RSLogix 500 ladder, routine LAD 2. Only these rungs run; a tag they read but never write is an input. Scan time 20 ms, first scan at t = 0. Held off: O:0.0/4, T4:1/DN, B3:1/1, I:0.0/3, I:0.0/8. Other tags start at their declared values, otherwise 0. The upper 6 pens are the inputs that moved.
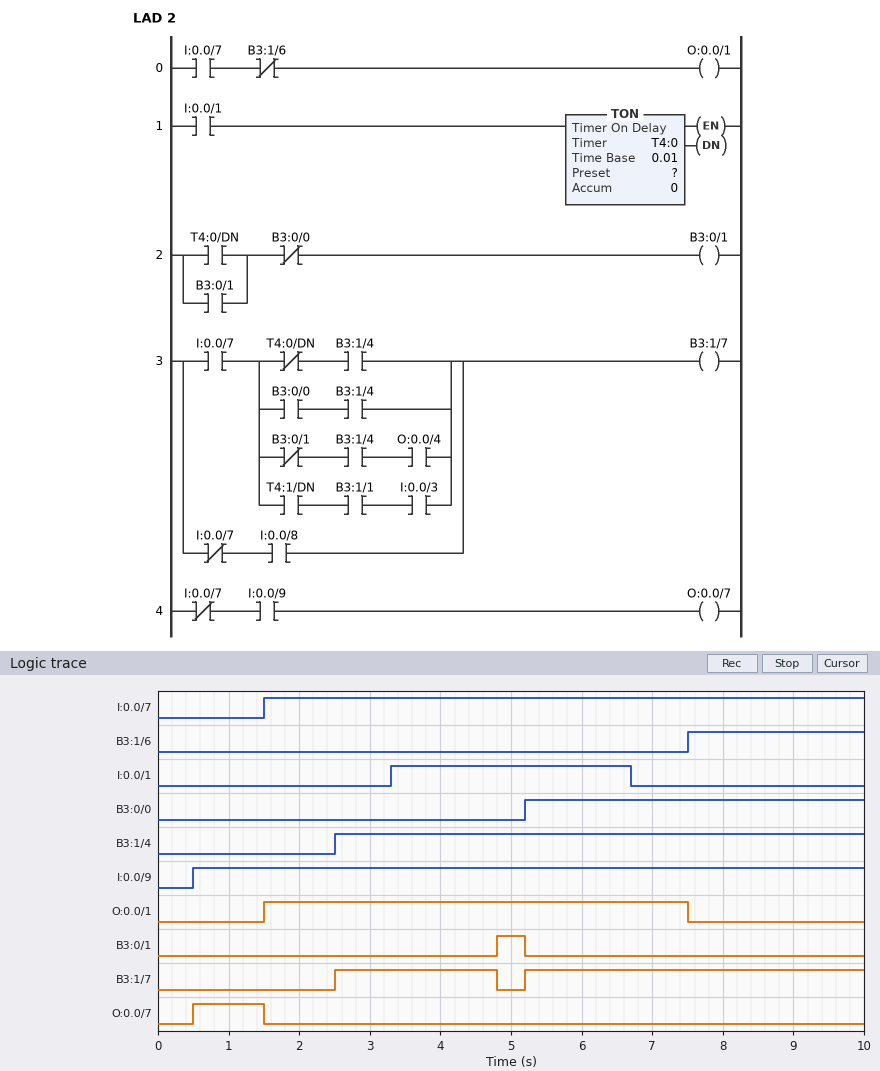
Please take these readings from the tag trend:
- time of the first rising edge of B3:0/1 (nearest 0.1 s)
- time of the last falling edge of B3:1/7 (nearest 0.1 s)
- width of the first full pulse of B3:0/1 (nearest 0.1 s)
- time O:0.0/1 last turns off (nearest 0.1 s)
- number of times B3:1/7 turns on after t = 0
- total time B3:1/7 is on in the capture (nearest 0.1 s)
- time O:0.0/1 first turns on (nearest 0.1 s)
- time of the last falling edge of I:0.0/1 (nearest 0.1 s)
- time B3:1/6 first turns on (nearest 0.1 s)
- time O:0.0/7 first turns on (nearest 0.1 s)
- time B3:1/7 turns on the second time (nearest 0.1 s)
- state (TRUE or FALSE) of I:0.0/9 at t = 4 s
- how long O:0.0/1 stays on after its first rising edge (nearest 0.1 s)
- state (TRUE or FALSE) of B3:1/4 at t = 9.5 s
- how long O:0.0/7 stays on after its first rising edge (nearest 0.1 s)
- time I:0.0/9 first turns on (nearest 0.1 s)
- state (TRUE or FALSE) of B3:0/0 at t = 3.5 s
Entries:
4.8 s
4.8 s
0.4 s
7.5 s
2
7.1 s
1.5 s
6.7 s
7.5 s
0.5 s
5.2 s
TRUE
6.0 s
TRUE
1.0 s
0.5 s
FALSE
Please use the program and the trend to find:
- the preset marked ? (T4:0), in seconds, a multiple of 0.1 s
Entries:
1.5 s
